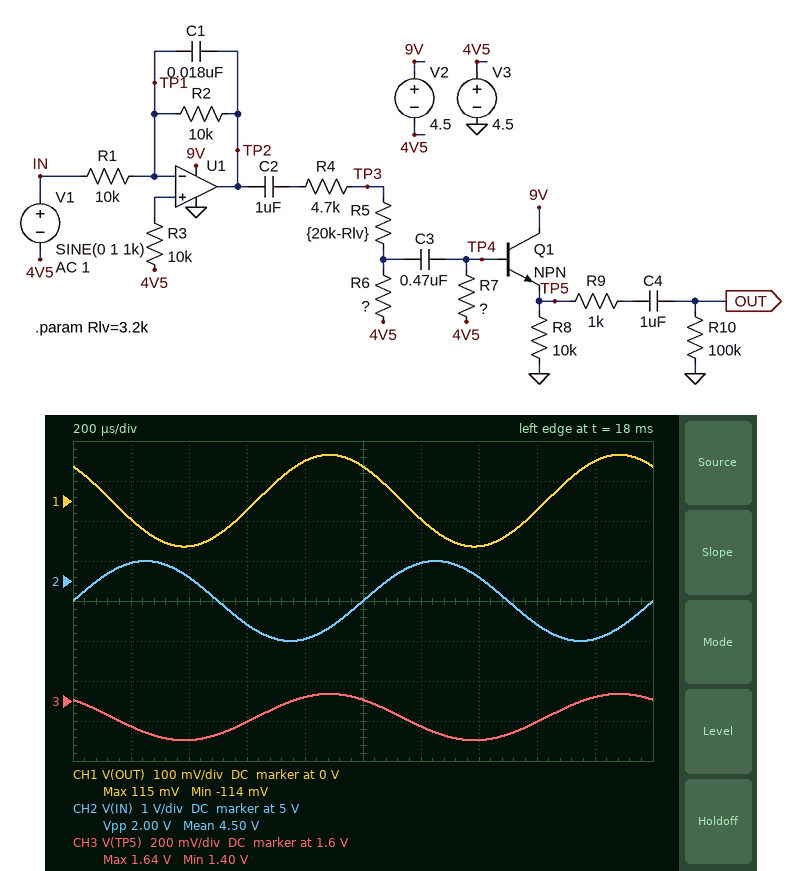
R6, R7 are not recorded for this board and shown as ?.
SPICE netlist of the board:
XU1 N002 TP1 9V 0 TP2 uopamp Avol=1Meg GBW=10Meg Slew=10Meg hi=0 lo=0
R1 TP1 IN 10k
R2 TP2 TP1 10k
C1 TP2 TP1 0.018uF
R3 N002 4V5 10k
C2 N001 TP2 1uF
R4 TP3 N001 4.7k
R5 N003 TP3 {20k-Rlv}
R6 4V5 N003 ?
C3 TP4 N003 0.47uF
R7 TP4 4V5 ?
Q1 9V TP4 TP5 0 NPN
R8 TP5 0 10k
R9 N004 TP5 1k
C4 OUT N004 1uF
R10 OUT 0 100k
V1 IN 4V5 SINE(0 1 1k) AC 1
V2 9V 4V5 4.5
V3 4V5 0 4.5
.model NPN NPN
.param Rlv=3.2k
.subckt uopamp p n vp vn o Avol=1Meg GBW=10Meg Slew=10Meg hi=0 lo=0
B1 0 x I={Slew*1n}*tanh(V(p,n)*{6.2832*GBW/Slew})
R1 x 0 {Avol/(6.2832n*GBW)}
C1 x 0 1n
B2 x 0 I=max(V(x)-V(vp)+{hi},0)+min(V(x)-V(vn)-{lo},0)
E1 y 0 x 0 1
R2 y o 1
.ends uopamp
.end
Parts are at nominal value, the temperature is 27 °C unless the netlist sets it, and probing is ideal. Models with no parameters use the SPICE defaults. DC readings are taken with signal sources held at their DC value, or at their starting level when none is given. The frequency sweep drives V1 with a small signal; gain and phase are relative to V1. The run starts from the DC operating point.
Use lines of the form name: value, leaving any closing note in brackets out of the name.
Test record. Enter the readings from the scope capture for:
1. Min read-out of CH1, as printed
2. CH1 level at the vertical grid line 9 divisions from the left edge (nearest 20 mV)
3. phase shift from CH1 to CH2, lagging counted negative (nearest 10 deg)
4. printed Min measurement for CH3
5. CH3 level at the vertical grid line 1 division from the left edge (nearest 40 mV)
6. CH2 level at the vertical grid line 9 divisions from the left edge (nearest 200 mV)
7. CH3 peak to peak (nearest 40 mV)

Min read-out of CH1, as printed: -114 mV
CH1 level at the vertical grid line 9 divisions from the left edge: 100 mV
phase shift from CH1 to CH2, lagging counted negative: -130 deg
printed Min measurement for CH3: 1.40 V
CH3 level at the vertical grid line 1 division from the left edge: 1.48 V
CH2 level at the vertical grid line 9 divisions from the left edge: 3.6 V
CH3 peak to peak: 240 mV
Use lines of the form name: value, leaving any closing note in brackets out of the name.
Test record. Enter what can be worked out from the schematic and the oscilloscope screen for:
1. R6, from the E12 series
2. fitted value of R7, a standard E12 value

R6, from the E12 series: 4.7 kΩ
fitted value of R7, a standard E12 value: 1.5 MΩ
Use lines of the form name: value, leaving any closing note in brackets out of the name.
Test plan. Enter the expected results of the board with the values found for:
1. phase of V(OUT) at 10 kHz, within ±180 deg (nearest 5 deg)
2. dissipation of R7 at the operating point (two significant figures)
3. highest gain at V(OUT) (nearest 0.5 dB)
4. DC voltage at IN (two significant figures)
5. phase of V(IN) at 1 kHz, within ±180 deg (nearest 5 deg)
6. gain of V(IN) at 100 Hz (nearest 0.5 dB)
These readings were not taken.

phase of V(OUT) at 10 kHz, within ±180 deg: 95 deg
dissipation of R7 at the operating point: 3.4 µW
highest gain at V(OUT): -15.5 dB
DC voltage at IN: 4.5 V
phase of V(IN) at 1 kHz, within ±180 deg: 0 deg
gain of V(IN) at 100 Hz: 0 dB
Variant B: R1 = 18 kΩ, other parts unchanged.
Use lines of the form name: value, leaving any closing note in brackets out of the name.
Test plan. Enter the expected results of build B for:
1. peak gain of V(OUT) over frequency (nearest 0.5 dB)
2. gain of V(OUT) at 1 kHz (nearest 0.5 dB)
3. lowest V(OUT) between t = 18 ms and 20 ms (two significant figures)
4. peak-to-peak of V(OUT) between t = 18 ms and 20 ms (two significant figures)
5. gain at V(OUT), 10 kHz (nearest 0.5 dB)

peak gain of V(OUT) over frequency: -20.5 dB
gain of V(OUT) at 1 kHz: -24.0 dB
lowest V(OUT) between t = 18 ms and 20 ms: -63 mV
peak-to-peak of V(OUT) between t = 18 ms and 20 ms: 130 mV
gain at V(OUT), 10 kHz: -41.5 dB
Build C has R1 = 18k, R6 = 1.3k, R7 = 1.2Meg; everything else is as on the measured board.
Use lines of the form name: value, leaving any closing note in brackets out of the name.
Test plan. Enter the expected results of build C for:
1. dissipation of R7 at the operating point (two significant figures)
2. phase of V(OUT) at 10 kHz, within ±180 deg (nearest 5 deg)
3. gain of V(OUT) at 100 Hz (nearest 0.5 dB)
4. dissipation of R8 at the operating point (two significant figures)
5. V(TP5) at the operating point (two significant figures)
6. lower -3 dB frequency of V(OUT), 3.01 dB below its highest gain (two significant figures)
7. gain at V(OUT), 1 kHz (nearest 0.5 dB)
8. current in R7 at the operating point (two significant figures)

dissipation of R7 at the operating point: 3.5 µW
phase of V(OUT) at 10 kHz, within ±180 deg: 95 deg
gain of V(OUT) at 100 Hz: -30.5 dB
dissipation of R8 at the operating point: 300 µW
V(TP5) at the operating point: 1.7 V
lower -3 dB frequency of V(OUT), 3.01 dB below its highest gain: 7.3 Hz
gain at V(OUT), 1 kHz: -34.0 dB
current in R7 at the operating point: 1.7 µA
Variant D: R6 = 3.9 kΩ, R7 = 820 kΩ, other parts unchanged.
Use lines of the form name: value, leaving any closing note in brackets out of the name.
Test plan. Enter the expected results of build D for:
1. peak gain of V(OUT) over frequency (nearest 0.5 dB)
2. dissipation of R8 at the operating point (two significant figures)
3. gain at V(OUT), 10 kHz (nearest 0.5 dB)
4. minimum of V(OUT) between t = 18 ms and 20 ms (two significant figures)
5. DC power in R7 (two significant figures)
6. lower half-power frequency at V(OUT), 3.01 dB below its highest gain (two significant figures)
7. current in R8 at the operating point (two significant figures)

peak gain of V(OUT) over frequency: -16.5 dB
dissipation of R8 at the operating point: 430 µW
gain at V(OUT), 10 kHz: -37.5 dB
minimum of V(OUT) between t = 18 ms and 20 ms: -98 mV
DC power in R7: 3.5 µW
lower half-power frequency at V(OUT), 3.01 dB below its highest gain: 6.6 Hz
current in R8 at the operating point: 210 µA
